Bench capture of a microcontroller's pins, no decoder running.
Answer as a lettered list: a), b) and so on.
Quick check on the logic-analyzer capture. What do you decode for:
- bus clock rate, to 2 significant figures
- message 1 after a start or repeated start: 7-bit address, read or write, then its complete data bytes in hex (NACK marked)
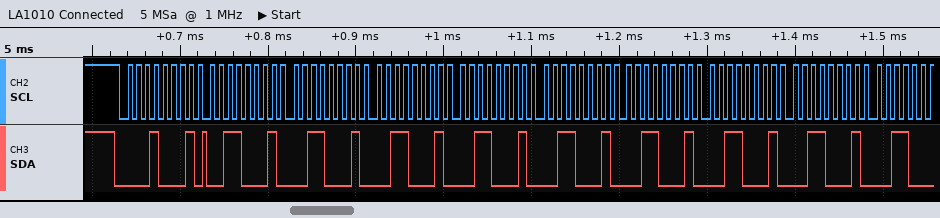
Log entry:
a) 100 kHz
b) 0x08 read: 31 31 31 31 31 31 31 31
